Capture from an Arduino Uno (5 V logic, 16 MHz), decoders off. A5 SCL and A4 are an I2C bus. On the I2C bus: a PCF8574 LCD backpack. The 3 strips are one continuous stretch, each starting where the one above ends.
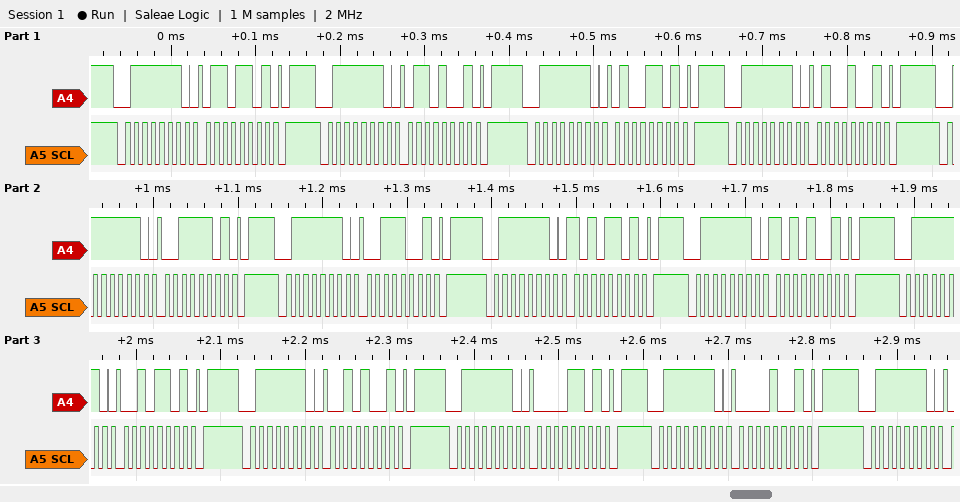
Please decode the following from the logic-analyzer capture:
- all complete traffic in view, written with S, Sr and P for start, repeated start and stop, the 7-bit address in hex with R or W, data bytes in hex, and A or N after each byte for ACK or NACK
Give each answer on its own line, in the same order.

S 3FW A 6D A P S 3FW A 69 A P S 3FW A 4D A P S 3FW A 49 A P S 3FW A 3D A P S 3FW A 39 A P S 3FW A AD A P S 3FW A A9 A P S 3FW A 2D A P S 3FW A 29 A P S 3FW A 0D A P S 3FW A 09 A P S 3FW A
